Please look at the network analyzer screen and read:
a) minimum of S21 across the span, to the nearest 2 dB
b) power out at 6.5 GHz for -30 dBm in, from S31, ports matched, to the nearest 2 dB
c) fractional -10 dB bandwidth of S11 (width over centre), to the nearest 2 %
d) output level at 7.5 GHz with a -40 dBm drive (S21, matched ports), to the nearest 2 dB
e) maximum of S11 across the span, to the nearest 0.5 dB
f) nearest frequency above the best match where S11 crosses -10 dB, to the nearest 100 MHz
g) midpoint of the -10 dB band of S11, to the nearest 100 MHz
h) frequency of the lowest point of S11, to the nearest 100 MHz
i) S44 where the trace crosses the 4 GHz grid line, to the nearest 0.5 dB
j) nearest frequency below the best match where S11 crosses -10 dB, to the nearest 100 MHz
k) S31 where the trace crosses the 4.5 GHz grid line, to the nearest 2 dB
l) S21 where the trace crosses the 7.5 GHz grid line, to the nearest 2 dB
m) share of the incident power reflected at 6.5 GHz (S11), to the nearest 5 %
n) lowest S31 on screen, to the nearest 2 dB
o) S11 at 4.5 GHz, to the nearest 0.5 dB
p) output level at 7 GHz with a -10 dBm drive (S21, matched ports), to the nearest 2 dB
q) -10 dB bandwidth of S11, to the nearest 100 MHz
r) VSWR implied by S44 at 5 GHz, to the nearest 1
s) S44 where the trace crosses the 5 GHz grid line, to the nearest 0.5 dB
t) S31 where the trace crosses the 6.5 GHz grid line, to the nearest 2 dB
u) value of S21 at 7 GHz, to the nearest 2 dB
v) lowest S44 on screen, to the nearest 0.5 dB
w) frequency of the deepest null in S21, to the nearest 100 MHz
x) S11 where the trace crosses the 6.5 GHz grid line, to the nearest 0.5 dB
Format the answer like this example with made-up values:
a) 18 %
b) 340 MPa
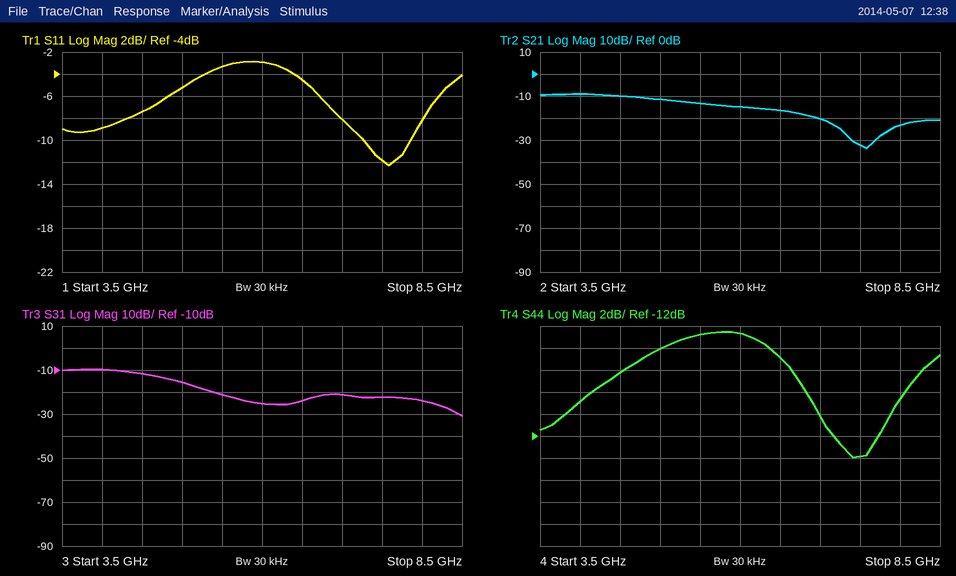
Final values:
a) -34 dB
b) -54 dBm
c) 8 %
d) -72 dBm
e) -3.0 dB
f) 7.9 GHz
g) 7.6 GHz
h) 7.6 GHz
i) -9.0 dB
j) 7.3 GHz
k) -12 dB
l) -32 dB
m) 35 %
n) -30 dB
o) -7.5 dB
p) -30 dBm
q) 600 MHz
r) 4
s) -4.0 dB
t) -24 dB
u) -20 dB
v) -14.0 dB
w) 7.6 GHz
x) -4.5 dB
